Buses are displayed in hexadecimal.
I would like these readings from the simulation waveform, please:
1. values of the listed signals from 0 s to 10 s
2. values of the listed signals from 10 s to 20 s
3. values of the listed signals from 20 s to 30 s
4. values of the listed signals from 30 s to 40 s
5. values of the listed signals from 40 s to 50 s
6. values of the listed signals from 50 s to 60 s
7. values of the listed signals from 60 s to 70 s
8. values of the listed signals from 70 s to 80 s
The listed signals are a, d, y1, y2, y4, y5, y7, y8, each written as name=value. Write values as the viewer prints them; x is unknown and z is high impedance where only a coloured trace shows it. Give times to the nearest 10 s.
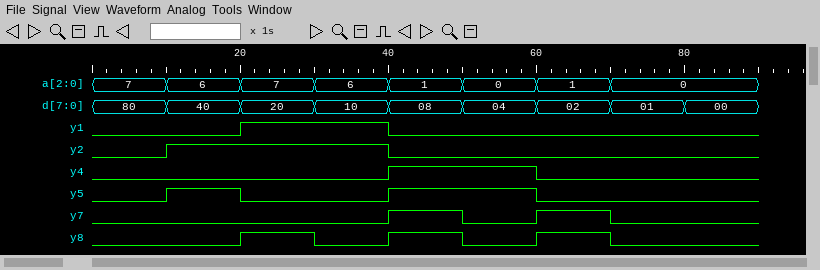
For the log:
a=7, d=80, y1=0, y2=0, y4=0, y5=0, y7=0, y8=0
a=6, d=40, y1=0, y2=1, y4=0, y5=1, y7=0, y8=0
a=7, d=20, y1=1, y2=1, y4=0, y5=0, y7=0, y8=1
a=6, d=10, y1=1, y2=1, y4=0, y5=0, y7=0, y8=0
a=1, d=08, y1=0, y2=0, y4=1, y5=1, y7=1, y8=1
a=0, d=04, y1=0, y2=0, y4=1, y5=1, y7=0, y8=0
a=1, d=02, y1=0, y2=0, y4=0, y5=0, y7=1, y8=1
a=0, d=01, y1=0, y2=0, y4=0, y5=0, y7=0, y8=0
